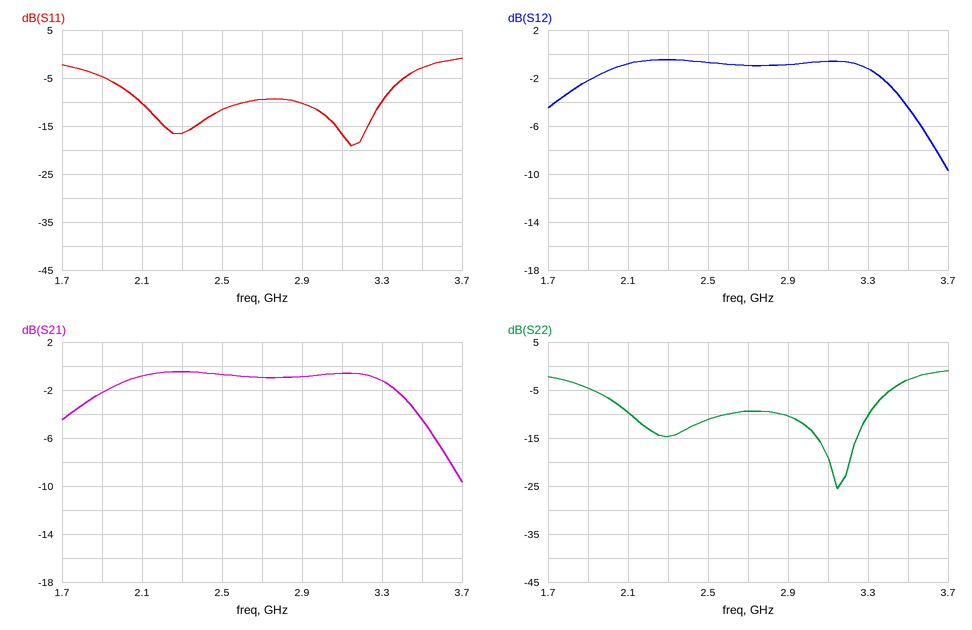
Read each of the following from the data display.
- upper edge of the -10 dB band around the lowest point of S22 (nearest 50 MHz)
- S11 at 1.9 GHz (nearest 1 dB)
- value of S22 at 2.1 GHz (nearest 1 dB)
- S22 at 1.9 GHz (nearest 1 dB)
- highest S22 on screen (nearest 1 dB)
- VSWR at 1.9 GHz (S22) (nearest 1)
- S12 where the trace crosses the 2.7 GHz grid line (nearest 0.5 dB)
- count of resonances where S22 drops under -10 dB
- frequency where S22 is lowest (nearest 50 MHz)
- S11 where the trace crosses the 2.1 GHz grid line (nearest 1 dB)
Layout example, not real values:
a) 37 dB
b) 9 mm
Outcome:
a) 3.30 GHz
b) -5 dB
c) -10 dB
d) -5 dB
e) -1 dB
f) 4
g) -1.0 dB
h) 2
i) 3.15 GHz
j) -10 dB
